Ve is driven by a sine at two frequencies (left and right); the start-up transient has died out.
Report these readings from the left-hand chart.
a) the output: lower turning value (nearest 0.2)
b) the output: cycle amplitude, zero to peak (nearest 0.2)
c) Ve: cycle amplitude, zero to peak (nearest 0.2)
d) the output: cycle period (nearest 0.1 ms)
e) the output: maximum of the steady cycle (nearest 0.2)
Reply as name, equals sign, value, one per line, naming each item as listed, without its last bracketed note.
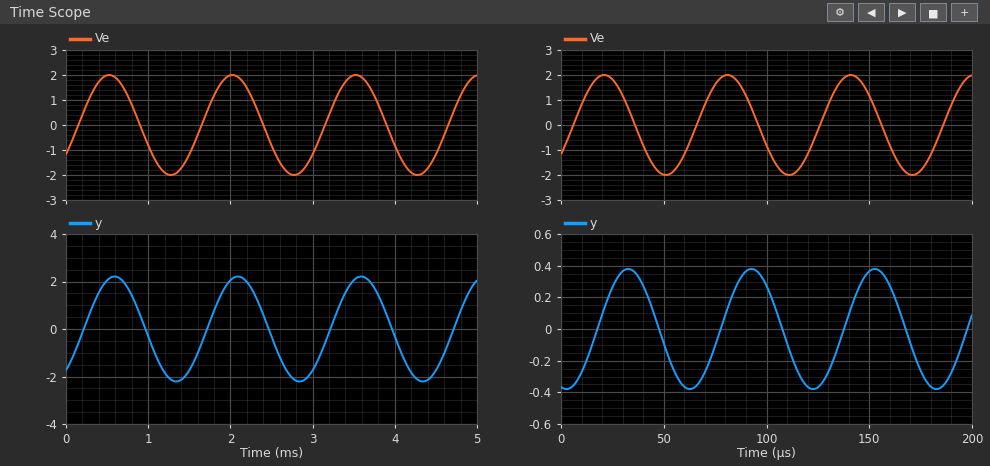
the output: lower turning value = -2.2
the output: cycle amplitude, zero to peak = 2.2
Ve: cycle amplitude, zero to peak = 2.0
the output: cycle period = 1.5 ms
the output: maximum of the steady cycle = 2.2
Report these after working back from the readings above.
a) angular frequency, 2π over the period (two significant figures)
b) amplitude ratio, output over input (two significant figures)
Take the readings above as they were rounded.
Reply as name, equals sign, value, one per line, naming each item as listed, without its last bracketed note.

angular frequency, 2π over the period = 4.2 rad/ms
amplitude ratio, output over input = 1.1
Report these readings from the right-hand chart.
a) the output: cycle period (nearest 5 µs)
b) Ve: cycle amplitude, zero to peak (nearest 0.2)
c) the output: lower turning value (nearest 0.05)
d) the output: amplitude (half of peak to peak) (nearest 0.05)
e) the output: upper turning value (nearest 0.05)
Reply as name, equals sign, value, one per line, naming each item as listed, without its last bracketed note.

the output: cycle period = 60 µs
Ve: cycle amplitude, zero to peak = 2.0
the output: lower turning value = -0.40
the output: amplitude (half of peak to peak) = 0.40
the output: upper turning value = 0.40
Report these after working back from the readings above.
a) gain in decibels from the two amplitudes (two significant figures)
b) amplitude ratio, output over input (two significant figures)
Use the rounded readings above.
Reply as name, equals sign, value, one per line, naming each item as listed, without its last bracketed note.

gain in decibels from the two amplitudes = -14 dB
amplitude ratio, output over input = 0.20
